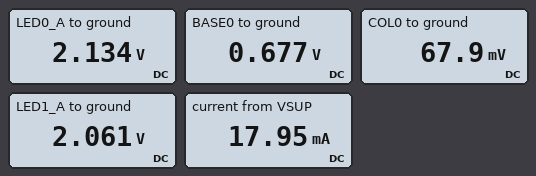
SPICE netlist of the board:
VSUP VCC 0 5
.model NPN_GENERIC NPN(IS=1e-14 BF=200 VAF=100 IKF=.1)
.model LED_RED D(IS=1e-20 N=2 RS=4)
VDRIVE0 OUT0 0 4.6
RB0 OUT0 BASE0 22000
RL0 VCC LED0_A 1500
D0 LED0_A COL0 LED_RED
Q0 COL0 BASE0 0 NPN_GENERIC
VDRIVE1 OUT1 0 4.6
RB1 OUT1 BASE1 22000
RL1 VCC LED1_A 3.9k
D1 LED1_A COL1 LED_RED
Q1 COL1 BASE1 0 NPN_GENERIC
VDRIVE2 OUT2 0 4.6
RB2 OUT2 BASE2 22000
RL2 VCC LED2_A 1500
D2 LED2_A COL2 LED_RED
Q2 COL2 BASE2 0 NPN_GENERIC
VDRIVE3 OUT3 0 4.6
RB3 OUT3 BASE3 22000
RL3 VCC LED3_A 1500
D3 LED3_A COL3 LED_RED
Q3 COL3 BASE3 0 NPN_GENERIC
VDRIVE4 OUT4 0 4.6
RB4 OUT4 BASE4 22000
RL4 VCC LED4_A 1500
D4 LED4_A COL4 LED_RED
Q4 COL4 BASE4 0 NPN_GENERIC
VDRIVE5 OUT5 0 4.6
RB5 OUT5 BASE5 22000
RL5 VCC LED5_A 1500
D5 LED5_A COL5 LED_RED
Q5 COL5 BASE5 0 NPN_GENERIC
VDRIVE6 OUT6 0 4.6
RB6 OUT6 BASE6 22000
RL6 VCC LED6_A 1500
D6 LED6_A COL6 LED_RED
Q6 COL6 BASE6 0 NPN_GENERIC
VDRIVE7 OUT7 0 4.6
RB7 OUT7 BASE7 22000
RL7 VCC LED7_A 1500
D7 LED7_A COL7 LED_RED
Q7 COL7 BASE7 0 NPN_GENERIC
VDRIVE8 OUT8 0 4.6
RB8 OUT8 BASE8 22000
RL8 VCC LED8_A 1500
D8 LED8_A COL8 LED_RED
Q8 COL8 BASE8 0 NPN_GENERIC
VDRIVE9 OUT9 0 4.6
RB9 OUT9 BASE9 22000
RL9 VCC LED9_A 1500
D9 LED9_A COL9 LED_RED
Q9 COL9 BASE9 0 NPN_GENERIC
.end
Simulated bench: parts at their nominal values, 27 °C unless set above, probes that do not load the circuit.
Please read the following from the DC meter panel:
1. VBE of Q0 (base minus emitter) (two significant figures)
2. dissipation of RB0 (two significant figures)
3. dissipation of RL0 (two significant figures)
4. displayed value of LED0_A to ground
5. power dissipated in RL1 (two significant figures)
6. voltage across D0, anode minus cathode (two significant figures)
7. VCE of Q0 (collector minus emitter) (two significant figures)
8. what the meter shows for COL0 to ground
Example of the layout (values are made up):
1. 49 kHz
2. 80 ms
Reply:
1. 680 mV
2. 700 µW
3. 5.5 mW
4. 2.134 V
5. 2.2 mW
6. 2.1 V
7. 68 mV
8. 67.9 mV
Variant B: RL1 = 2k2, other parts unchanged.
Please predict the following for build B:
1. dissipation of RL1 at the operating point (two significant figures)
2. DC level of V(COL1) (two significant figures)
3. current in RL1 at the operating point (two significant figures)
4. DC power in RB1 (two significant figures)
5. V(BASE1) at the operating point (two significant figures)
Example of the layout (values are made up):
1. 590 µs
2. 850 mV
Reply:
1. 3.8 mW
2. 59 mV
3. 1.3 mA
4. 700 µW
5. 670 mV
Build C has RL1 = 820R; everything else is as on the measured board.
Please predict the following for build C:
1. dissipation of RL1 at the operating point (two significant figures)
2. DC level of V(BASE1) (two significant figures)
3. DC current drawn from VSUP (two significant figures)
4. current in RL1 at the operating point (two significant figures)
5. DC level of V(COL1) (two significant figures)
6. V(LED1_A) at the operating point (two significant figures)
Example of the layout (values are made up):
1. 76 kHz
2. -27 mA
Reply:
1. 9.7 mW
2. 690 mV
3. 21 mA
4. 3.4 mA
5. 83 mV
6. 2.2 V
